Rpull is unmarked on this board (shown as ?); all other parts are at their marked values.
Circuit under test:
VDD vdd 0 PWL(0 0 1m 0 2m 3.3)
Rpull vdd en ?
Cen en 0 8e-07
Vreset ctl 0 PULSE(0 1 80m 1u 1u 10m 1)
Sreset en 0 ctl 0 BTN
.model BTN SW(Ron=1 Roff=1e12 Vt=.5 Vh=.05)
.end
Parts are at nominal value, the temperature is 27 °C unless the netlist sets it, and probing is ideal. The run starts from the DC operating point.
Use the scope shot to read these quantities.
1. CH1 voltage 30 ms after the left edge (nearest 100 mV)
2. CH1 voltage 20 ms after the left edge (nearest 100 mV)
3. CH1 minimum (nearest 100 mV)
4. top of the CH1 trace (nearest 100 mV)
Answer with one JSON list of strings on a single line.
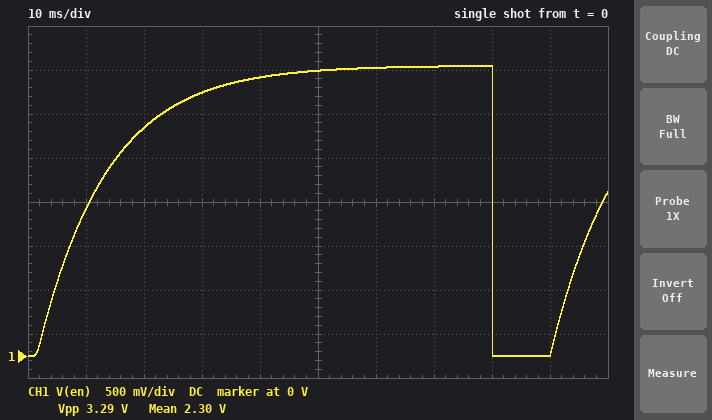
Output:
["3.0 V", "2.6 V", "0 V", "3.3 V"]
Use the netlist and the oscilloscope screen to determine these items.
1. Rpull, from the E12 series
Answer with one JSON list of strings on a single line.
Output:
["15 kΩ"]
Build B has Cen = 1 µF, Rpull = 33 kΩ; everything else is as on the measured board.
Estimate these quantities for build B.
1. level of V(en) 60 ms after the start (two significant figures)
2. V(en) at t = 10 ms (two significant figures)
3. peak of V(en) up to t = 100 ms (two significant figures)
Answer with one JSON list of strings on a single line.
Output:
["2.7 V", "750 mV", "3.0 V"]
